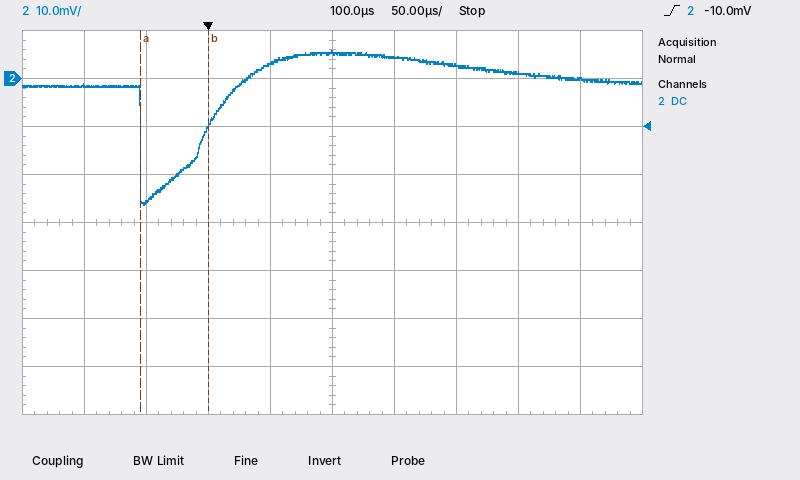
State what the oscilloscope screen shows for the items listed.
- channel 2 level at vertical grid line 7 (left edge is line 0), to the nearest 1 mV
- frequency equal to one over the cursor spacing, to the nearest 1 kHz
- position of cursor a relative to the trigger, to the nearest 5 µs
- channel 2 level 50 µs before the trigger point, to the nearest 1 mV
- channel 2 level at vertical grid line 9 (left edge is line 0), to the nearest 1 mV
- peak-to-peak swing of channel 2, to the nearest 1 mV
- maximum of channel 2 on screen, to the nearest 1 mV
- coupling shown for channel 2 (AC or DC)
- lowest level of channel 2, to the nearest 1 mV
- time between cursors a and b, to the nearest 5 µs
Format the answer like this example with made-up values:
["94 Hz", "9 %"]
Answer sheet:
["3 mV", "18 kHz", "-55 µs", "-26 mV", "0 mV", "32 mV", "6 mV", "DC", "-26 mV", "55 µs"]
